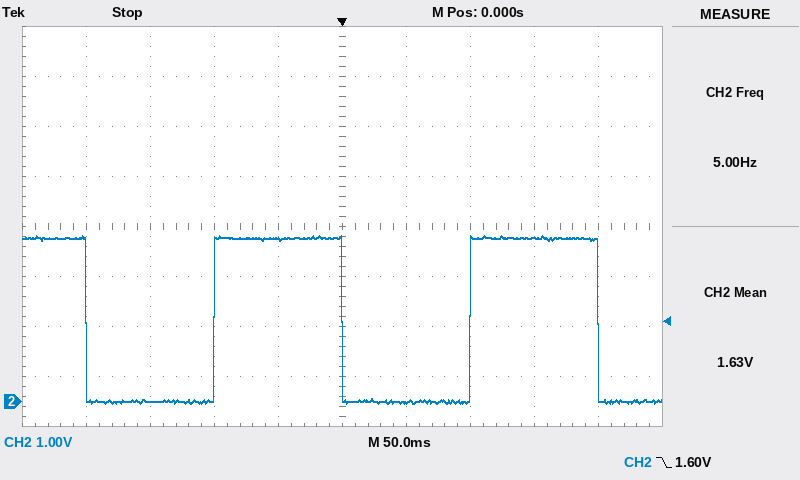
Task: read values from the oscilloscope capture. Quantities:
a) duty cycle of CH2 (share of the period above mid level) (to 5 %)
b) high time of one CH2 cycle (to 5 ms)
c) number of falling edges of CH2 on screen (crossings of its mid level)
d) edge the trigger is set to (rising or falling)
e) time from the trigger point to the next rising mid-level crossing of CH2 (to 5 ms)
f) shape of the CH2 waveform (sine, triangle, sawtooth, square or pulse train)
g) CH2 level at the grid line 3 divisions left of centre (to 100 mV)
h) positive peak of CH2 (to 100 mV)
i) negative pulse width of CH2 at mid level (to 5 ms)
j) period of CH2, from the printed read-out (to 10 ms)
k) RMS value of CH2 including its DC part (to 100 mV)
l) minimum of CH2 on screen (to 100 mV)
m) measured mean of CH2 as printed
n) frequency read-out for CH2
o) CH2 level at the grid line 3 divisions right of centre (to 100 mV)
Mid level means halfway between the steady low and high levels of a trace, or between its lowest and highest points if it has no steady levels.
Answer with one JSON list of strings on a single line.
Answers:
["50 %", "100 ms", "3", "falling", "100 ms", "square", "0.0 V", "3.3 V", "100 ms", "200 ms", "2.3 V", "0.0 V", "1.63 V", "5.00 Hz", "3.3 V"]
